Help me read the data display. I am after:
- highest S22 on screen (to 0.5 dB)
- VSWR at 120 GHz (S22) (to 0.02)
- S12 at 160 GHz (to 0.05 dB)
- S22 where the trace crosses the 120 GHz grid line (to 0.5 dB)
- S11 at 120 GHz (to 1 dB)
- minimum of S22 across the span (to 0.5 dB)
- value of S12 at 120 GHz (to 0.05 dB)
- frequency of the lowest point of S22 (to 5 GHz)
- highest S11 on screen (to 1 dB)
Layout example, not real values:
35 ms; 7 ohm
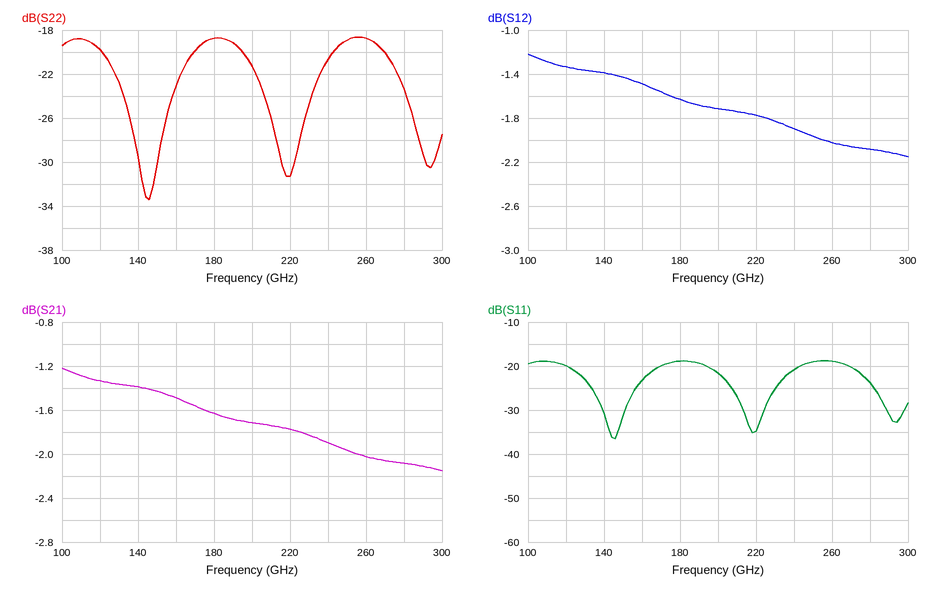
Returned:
-18.5 dB; 1.22; -1.50 dB; -20.0 dB; -20 dB; -33.5 dB; -1.35 dB; 145 GHz; -19 dB
